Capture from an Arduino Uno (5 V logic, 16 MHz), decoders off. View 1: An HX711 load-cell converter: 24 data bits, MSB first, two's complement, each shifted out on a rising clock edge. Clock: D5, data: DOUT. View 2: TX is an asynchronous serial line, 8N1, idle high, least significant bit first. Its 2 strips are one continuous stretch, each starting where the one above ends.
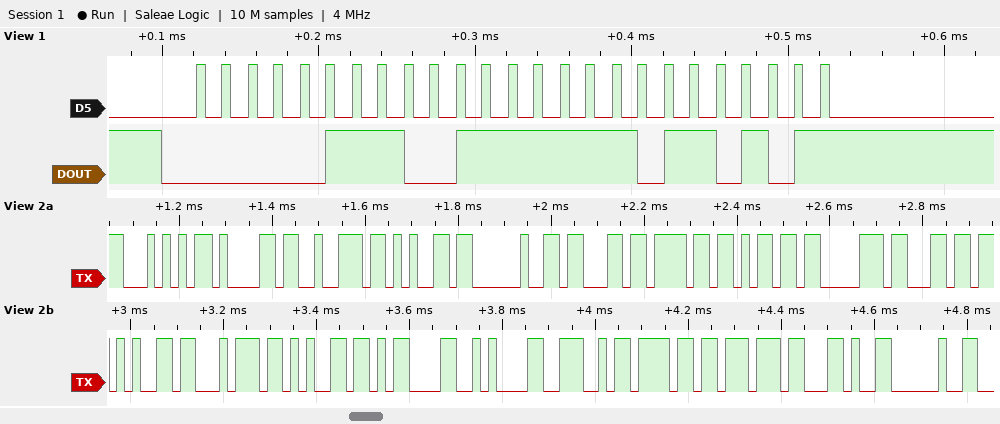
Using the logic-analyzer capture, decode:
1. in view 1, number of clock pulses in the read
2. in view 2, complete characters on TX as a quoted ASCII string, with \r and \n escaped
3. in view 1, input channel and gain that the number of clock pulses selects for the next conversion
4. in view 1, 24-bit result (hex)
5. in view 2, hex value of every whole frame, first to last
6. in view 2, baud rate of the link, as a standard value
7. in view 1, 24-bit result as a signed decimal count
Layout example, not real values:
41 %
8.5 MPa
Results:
25
"Tare complete\r\nNow, "
channel A, gain 128
0x073FB5
54 61 72 65 20 63 6F 6D 70 6C 65 74 65 0D 0A 4E 6F 77 2C 20
57600 baud
475061
